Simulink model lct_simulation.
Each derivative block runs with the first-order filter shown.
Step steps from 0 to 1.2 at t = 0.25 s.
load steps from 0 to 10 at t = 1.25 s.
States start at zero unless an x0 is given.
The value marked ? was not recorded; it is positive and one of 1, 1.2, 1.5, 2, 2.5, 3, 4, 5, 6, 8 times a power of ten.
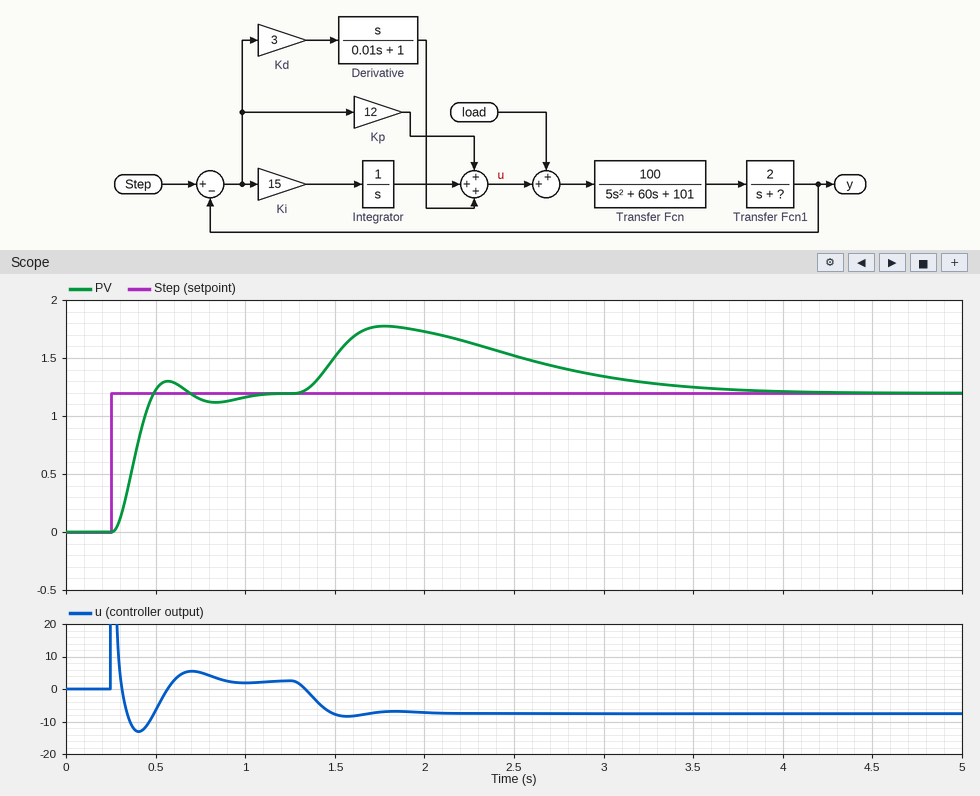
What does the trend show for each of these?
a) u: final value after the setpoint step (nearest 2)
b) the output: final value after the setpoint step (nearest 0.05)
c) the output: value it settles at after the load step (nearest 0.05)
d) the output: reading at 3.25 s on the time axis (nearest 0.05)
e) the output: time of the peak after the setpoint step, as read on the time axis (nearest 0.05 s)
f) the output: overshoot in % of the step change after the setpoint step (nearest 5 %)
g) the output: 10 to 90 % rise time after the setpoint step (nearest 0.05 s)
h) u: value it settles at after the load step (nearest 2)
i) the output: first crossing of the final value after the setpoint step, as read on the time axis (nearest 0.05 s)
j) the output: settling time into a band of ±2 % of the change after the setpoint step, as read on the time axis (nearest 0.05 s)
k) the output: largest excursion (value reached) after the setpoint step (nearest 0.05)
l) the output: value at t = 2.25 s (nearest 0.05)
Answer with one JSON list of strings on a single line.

["2", "1.20", "1.20", "1.30", "0.55 s", "10 %", "0.15 s", "-8", "0.50 s", "1.05 s", "1.30", "1.65"]
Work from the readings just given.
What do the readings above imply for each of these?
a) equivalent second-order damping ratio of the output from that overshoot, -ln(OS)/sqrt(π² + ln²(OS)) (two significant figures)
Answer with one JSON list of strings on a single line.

["0.59"]
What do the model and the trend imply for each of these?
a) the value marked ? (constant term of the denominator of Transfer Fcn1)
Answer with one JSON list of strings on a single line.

["4"]
